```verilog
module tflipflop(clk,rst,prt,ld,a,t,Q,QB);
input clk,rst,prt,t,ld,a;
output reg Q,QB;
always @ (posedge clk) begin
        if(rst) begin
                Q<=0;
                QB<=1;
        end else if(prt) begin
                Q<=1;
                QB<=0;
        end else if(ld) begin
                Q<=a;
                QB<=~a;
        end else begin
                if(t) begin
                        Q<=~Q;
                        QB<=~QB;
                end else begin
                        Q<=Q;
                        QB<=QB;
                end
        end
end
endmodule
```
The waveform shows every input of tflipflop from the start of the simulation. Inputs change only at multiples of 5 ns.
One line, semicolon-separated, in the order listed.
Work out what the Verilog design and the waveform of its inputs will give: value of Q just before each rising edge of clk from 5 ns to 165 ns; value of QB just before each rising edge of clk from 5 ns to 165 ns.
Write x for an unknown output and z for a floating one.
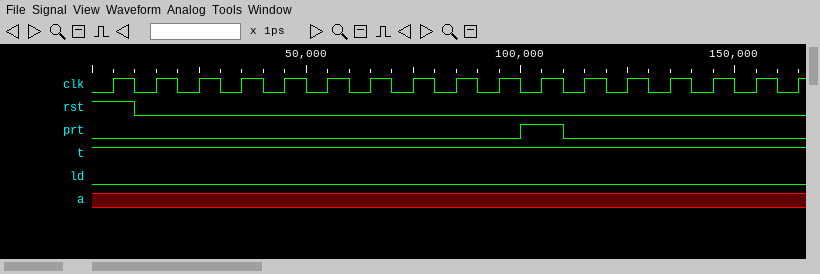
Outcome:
x 0 1 0 1 0 1 0 1 0 1 1 0 1 0 1 0; x 1 0 1 0 1 0 1 0 1 0 0 1 0 1 0 1
